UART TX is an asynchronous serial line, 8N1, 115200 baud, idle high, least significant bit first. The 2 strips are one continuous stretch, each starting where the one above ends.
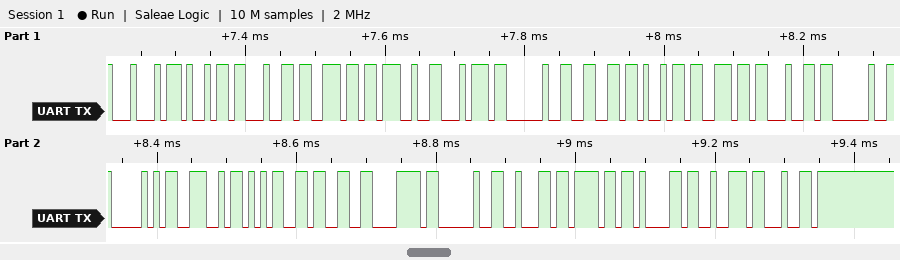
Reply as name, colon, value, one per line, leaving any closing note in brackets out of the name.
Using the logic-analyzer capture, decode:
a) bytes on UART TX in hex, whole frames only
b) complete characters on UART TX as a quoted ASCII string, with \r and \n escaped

bytes on UART TX in hex, whole frames only: 0x44 0x69 0x64 0x6E 0x27 0x74 0x20 0x66 0x69 0x6E 0x64 0x20 0x50 0x4E 0x35 0x33 0x78 0x20 0x62 0x6F 0x61 0x72 0x64
complete characters on UART TX as a quoted ASCII string, with \r and \n escaped: "Didn't find PN53x board"
